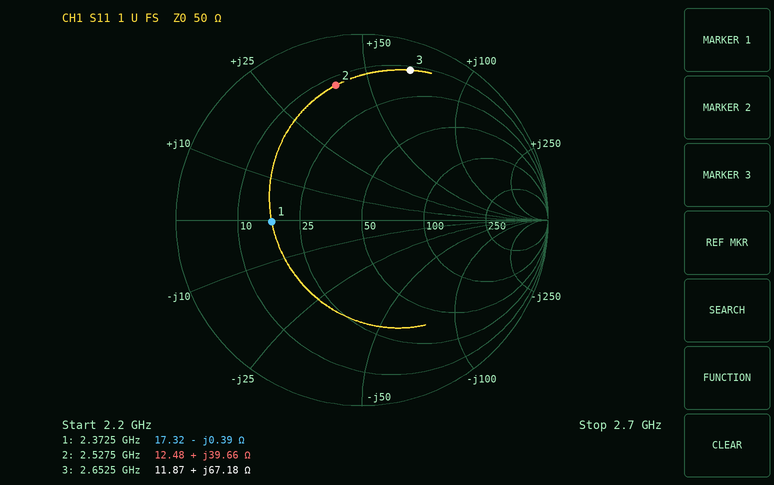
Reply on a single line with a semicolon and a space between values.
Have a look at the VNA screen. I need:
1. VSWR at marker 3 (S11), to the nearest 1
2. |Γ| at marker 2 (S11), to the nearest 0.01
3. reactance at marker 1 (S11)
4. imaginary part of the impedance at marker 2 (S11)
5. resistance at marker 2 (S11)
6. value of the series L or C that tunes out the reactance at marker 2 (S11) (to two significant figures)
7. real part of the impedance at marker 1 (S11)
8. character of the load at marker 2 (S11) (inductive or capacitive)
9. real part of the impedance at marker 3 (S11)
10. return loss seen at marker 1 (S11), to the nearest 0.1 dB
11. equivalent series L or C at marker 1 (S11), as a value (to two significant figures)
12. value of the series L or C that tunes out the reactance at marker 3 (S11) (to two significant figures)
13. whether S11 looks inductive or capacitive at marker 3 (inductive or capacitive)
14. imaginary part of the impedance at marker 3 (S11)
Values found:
12; 0.74; -0.39 Ω; +39.66 Ω; 12.48 Ω; 1.6 pF; 17.32 Ω; inductive; 11.87 Ω; 6.3 dB; 170 pF; 890 fF; inductive; +67.18 Ω
